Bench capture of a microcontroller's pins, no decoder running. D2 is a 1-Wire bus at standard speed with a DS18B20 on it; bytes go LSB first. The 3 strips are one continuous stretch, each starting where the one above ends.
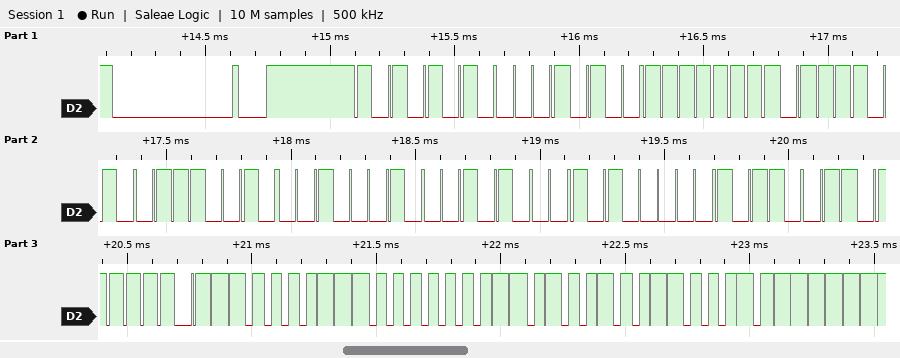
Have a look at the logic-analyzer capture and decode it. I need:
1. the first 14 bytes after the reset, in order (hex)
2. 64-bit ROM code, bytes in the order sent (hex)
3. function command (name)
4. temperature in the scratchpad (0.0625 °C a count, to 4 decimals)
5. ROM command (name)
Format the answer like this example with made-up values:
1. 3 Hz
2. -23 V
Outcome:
1. 55 28 FF 5E 4E 44 14 05 CD BE C3 01 4B 46
2. 28 FF 5E 4E 44 14 05 CD
3. Read Scratchpad
4. 28.1875 °C
5. Match ROM
